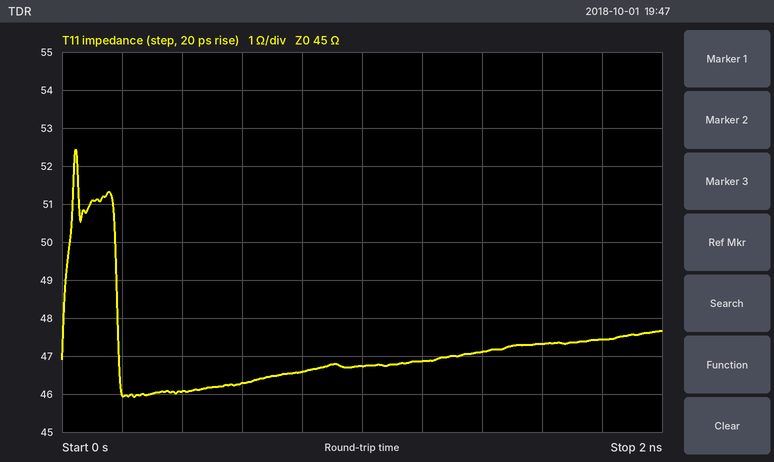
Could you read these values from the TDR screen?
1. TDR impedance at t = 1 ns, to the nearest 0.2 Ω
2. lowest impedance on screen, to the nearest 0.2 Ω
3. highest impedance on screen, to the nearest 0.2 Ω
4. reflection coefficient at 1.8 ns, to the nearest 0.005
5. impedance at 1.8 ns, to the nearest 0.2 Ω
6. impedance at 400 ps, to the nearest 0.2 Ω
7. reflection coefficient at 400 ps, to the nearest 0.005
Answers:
46.8 Ω
46.0 Ω
52.4 Ω
+0.025
47.4 Ω
46.0 Ω
+0.010
